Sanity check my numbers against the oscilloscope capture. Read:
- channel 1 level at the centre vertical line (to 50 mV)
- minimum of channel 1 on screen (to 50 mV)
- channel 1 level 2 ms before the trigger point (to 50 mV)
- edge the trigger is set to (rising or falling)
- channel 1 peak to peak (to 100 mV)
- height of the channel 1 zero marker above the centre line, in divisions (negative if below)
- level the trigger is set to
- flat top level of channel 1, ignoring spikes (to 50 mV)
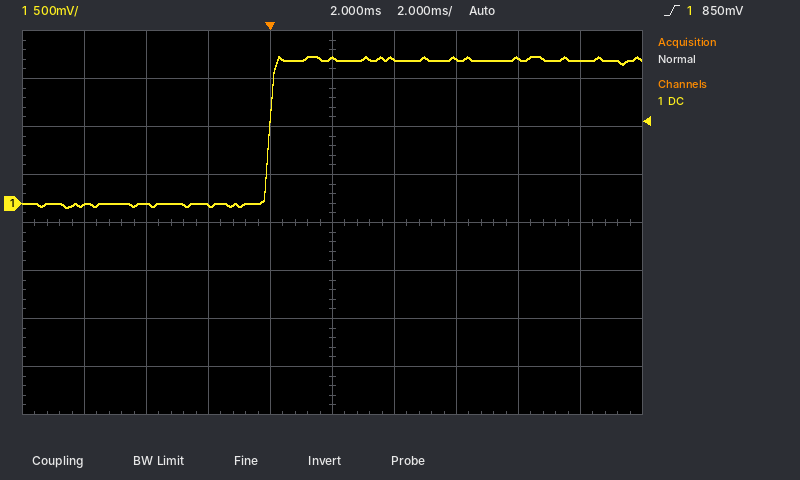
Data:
1.50 V
-50 mV
0 mV
rising
1.60 V
+0.4 div
850 mV
1.50 V
